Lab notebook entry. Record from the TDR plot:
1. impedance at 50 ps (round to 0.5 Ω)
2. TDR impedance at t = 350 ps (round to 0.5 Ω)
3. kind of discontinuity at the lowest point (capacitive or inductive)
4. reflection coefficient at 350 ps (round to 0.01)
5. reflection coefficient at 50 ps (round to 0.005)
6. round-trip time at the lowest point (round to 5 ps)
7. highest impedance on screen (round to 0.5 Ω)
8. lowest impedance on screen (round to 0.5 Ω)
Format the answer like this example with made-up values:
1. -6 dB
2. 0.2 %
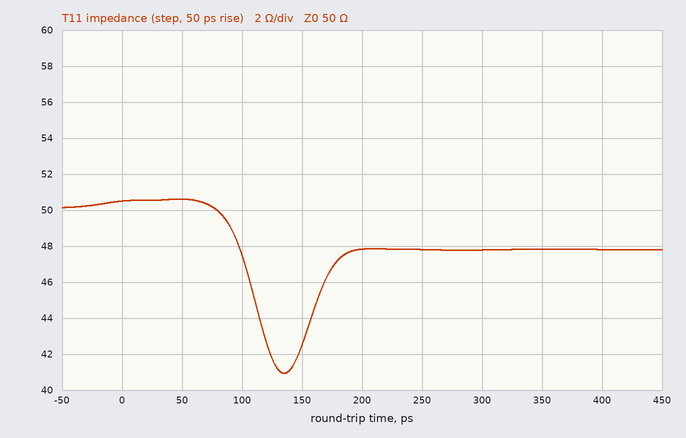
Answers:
1. 50.5 Ω
2. 48.0 Ω
3. capacitive
4. -0.02
5. +0.005
6. 135 ps
7. 50.5 Ω
8. 41.0 Ω
